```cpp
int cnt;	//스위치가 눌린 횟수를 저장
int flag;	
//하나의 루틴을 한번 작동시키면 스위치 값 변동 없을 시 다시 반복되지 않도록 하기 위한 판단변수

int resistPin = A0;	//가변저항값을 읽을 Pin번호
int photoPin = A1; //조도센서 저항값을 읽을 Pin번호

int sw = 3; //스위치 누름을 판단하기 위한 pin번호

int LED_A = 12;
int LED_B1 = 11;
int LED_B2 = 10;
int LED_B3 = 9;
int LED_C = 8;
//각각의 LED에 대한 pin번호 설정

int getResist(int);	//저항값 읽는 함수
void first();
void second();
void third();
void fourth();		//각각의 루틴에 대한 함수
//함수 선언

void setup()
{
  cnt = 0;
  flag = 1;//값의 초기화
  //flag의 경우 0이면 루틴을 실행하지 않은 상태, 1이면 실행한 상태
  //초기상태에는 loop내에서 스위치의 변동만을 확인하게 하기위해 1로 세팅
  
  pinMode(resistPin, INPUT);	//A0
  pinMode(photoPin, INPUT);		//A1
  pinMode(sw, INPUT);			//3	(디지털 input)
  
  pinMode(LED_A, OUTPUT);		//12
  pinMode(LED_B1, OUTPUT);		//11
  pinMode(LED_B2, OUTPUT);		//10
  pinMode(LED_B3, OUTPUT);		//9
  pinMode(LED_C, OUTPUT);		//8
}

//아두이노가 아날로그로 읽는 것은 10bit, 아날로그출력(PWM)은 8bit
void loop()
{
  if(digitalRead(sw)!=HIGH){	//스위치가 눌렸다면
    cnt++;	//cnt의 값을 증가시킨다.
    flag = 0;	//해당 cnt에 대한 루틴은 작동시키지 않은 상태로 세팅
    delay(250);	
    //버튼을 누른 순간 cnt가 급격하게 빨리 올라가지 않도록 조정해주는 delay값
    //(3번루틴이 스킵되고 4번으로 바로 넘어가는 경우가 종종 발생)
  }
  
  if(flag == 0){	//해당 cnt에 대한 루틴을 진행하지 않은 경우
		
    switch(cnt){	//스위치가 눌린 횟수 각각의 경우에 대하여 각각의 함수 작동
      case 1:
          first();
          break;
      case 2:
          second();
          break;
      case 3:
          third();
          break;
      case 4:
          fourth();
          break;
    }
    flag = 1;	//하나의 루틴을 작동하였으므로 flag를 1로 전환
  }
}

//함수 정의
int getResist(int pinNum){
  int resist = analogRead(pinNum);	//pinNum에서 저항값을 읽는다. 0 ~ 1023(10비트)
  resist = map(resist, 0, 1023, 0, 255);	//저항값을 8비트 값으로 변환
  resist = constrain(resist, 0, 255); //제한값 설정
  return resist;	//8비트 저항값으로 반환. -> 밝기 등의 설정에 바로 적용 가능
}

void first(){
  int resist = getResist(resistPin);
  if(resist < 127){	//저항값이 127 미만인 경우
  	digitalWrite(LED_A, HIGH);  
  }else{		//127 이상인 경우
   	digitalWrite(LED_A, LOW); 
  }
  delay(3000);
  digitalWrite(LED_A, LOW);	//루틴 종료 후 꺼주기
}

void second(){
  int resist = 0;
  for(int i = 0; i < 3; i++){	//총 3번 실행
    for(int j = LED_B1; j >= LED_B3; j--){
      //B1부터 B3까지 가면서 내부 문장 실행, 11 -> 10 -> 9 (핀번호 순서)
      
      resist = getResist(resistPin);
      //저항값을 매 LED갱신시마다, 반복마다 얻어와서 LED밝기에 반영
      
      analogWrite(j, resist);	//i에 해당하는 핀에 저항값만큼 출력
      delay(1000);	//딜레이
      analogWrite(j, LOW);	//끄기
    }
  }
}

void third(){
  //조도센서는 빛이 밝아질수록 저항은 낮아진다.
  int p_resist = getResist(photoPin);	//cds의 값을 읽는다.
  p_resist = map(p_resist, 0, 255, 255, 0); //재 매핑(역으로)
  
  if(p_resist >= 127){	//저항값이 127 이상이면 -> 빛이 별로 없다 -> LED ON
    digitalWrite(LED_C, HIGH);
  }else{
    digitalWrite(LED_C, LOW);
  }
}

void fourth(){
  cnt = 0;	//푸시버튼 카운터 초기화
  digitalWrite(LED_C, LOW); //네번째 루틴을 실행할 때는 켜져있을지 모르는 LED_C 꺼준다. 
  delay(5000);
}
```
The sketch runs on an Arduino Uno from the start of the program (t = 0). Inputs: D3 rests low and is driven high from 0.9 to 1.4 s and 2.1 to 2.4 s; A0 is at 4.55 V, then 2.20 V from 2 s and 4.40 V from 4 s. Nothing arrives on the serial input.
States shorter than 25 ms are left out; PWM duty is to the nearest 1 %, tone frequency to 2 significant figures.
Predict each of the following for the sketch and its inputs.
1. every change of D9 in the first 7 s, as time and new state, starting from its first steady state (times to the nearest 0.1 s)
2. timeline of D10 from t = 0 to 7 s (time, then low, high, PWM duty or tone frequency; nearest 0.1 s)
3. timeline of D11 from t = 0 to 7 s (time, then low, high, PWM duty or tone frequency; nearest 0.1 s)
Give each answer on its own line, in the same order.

0 s low; 5.5 s PWM 88 %; 6.5 s low
0 s low; 4.5 s PWM 88 %; 5.5 s low
0 s low; 3.5 s PWM 44 %; 4.5 s low; 6.5 s PWM 88 %
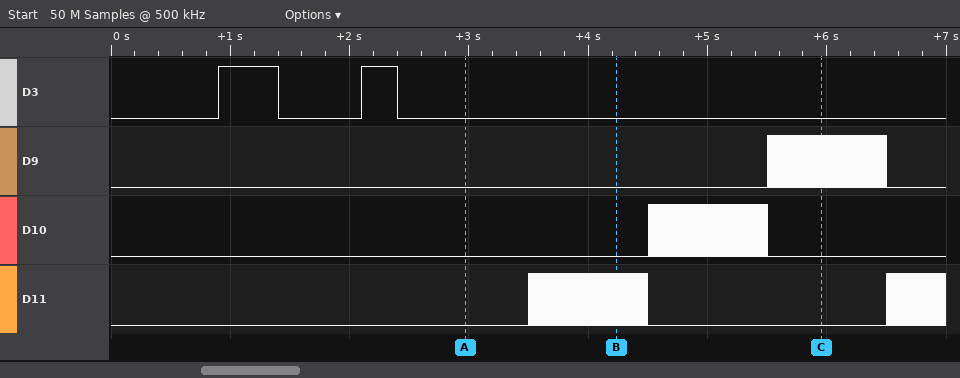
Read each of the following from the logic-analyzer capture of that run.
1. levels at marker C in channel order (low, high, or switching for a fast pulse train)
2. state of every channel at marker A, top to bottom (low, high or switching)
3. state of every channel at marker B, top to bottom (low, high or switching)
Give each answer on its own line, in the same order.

D3 low, D9 switching, D10 low, D11 low
D3 low, D9 low, D10 low, D11 low
D3 low, D9 low, D10 low, D11 switching
